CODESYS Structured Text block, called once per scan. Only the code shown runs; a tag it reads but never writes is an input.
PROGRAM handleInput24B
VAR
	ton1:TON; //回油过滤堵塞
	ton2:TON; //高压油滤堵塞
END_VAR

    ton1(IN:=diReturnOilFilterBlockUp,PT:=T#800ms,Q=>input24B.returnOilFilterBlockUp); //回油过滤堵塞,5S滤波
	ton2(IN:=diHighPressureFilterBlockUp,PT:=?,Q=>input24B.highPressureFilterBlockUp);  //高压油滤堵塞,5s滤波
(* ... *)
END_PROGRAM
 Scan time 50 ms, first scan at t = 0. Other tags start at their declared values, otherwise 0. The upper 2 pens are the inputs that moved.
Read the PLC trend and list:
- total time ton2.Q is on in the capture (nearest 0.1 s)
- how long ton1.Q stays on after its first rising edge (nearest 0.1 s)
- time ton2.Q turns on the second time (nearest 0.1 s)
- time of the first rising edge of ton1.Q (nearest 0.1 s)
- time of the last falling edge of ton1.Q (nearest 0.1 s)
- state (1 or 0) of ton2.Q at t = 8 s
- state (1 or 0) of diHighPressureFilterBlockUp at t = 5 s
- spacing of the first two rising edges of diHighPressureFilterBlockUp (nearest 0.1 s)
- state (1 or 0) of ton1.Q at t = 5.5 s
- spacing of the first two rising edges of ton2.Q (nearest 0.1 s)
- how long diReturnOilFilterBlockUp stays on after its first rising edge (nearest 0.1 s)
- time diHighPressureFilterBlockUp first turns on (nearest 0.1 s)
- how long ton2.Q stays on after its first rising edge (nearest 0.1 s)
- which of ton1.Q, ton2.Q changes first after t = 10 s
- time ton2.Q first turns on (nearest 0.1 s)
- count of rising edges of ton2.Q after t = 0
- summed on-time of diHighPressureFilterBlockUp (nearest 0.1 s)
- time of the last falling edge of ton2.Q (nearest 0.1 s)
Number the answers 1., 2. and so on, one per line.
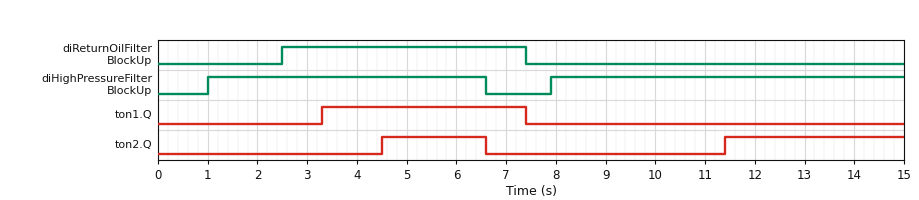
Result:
1. 5.7 s
2. 4.1 s
3. 11.4 s
4. 3.3 s
5. 7.4 s
6. 0
7. 1
8. 6.9 s
9. 1
10. 6.9 s
11. 4.9 s
12. 1.0 s
13. 2.1 s
14. ton2.Q
15. 4.5 s
16. 2
17. 12.7 s
18. 6.6 s
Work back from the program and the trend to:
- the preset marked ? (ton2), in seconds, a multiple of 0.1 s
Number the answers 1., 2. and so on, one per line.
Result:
1. 3.5 s
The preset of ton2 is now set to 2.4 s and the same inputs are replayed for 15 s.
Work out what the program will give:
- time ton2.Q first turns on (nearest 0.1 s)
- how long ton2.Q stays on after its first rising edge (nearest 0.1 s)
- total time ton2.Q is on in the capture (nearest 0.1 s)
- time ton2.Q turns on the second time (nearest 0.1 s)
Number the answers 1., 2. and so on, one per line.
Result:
1. 3.4 s
2. 3.2 s
3. 7.9 s
4. 10.3 s
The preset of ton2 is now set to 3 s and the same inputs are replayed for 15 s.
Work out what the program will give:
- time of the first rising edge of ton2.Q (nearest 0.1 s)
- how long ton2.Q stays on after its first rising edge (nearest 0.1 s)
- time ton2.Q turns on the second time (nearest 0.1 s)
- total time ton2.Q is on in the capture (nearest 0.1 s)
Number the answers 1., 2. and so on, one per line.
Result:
1. 4.0 s
2. 2.6 s
3. 10.9 s
4. 6.7 s
